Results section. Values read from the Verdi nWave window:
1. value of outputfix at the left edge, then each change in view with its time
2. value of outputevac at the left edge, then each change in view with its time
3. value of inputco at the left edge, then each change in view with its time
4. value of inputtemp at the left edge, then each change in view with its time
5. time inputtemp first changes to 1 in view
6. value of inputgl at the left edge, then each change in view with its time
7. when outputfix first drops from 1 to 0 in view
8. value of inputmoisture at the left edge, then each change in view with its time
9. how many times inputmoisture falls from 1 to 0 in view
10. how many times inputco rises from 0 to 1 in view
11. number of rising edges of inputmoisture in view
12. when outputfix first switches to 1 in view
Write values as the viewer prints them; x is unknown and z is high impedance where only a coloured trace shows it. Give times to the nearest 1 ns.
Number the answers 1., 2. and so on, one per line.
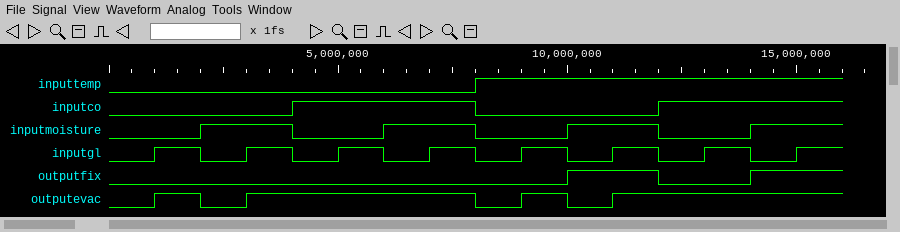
1. 0, 1 at 10 ns, 0 at 12 ns, 1 at 14 ns
2. 0, 1 at 1 ns, 0 at 2 ns, 1 at 3 ns, 0 at 8 ns, 1 at 9 ns, 0 at 10 ns, 1 at 11 ns
3. 0, 1 at 4 ns, 0 at 8 ns, 1 at 12 ns
4. 0, 1 at 8 ns
5. 8 ns
6. 0, 1 at 1 ns, 0 at 2 ns, 1 at 3 ns, 0 at 4 ns, 1 at 5 ns, 0 at 6 ns, 1 at 7 ns, 0 at 8 ns, 1 at 9 ns, 0 at 10 ns, 1 at 11 ns, 0 at 12 ns, 1 at 13 ns, 0 at 14 ns, 1 at 15 ns
7. 12 ns
8. 0, 1 at 2 ns, 0 at 4 ns, 1 at 6 ns, 0 at 8 ns, 1 at 10 ns, 0 at 12 ns, 1 at 14 ns
9. 3
10. 2
11. 4
12. 10 ns
